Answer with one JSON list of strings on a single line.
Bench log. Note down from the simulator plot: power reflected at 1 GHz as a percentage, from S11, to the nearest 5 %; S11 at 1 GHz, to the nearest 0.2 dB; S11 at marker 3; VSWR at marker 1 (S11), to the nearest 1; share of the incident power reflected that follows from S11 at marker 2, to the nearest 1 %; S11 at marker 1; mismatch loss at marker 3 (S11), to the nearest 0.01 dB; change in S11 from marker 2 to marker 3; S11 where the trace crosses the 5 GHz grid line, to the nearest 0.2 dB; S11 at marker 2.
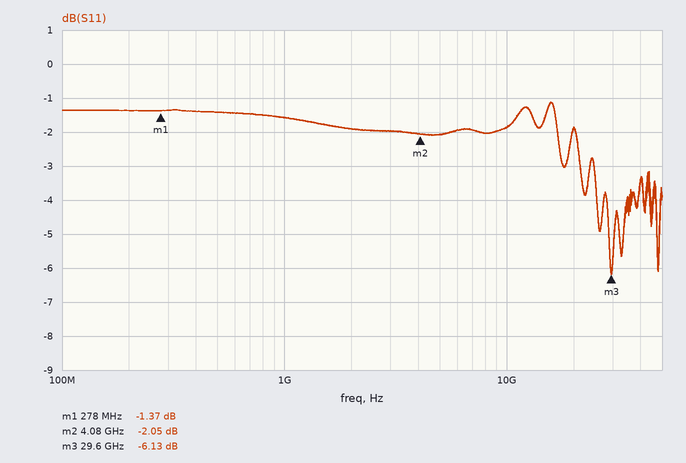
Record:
["70 %", "-1.6 dB", "-6.13 dB", "13", "62 %", "-1.37 dB", "1.21 dB", "-4.08 dB", "-2.0 dB", "-2.05 dB"]
